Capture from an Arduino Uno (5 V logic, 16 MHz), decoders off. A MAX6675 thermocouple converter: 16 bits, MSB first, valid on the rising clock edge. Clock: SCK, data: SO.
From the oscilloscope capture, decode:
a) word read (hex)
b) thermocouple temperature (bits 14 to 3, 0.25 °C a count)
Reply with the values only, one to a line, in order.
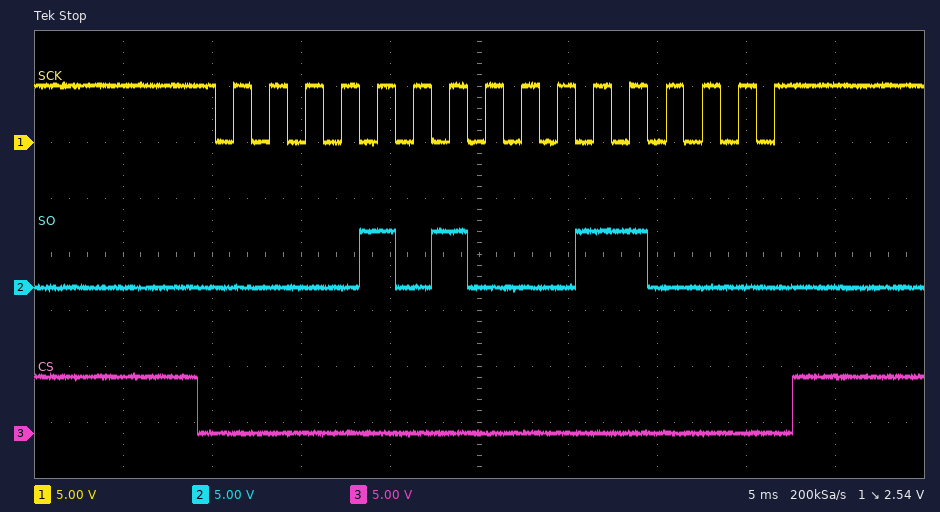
0x0A30
81.50 °C
